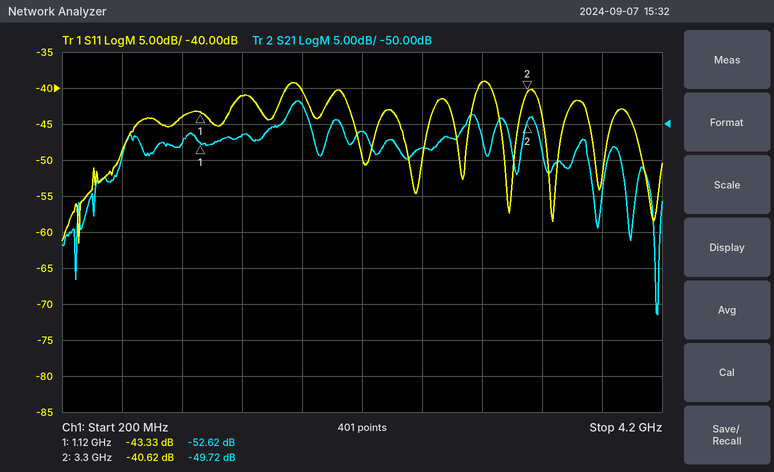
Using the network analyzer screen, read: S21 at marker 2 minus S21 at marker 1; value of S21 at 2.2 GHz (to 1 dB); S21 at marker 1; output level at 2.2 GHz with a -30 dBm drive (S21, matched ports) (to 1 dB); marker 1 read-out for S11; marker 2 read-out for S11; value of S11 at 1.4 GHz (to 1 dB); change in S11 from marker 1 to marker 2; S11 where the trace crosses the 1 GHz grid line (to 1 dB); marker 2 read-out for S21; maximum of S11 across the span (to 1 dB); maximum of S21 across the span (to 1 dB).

2.90 dB
-51 dB
-52.62 dB
-81 dBm
-43.33 dB
-40.62 dB
-41 dB
2.71 dB
-44 dB
-49.72 dB
-39 dB
-47 dB
